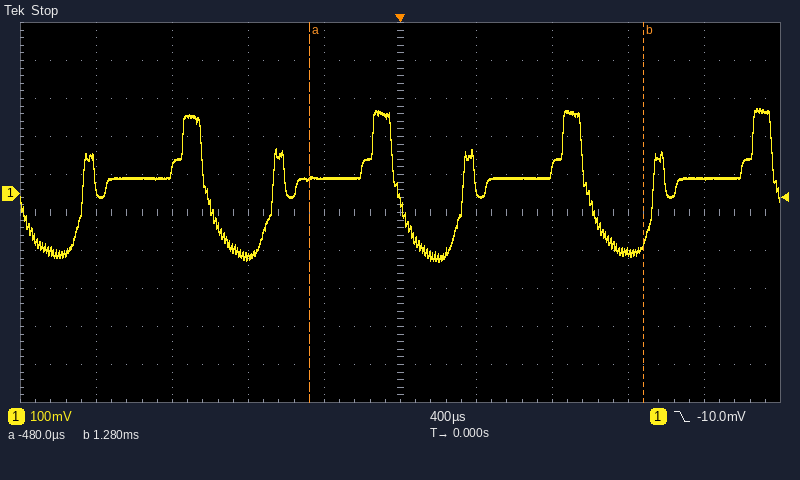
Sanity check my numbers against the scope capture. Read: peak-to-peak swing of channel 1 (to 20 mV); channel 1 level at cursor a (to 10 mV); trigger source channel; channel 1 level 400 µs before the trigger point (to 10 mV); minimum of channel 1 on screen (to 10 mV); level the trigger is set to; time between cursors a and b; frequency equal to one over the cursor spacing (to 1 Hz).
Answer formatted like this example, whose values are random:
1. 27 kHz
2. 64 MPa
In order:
1. 400 mV
2. 40 mV
3. channel 1
4. 40 mV
5. -180 mV
6. -10.0 mV
7. 1.76 ms
8. 568 Hz
